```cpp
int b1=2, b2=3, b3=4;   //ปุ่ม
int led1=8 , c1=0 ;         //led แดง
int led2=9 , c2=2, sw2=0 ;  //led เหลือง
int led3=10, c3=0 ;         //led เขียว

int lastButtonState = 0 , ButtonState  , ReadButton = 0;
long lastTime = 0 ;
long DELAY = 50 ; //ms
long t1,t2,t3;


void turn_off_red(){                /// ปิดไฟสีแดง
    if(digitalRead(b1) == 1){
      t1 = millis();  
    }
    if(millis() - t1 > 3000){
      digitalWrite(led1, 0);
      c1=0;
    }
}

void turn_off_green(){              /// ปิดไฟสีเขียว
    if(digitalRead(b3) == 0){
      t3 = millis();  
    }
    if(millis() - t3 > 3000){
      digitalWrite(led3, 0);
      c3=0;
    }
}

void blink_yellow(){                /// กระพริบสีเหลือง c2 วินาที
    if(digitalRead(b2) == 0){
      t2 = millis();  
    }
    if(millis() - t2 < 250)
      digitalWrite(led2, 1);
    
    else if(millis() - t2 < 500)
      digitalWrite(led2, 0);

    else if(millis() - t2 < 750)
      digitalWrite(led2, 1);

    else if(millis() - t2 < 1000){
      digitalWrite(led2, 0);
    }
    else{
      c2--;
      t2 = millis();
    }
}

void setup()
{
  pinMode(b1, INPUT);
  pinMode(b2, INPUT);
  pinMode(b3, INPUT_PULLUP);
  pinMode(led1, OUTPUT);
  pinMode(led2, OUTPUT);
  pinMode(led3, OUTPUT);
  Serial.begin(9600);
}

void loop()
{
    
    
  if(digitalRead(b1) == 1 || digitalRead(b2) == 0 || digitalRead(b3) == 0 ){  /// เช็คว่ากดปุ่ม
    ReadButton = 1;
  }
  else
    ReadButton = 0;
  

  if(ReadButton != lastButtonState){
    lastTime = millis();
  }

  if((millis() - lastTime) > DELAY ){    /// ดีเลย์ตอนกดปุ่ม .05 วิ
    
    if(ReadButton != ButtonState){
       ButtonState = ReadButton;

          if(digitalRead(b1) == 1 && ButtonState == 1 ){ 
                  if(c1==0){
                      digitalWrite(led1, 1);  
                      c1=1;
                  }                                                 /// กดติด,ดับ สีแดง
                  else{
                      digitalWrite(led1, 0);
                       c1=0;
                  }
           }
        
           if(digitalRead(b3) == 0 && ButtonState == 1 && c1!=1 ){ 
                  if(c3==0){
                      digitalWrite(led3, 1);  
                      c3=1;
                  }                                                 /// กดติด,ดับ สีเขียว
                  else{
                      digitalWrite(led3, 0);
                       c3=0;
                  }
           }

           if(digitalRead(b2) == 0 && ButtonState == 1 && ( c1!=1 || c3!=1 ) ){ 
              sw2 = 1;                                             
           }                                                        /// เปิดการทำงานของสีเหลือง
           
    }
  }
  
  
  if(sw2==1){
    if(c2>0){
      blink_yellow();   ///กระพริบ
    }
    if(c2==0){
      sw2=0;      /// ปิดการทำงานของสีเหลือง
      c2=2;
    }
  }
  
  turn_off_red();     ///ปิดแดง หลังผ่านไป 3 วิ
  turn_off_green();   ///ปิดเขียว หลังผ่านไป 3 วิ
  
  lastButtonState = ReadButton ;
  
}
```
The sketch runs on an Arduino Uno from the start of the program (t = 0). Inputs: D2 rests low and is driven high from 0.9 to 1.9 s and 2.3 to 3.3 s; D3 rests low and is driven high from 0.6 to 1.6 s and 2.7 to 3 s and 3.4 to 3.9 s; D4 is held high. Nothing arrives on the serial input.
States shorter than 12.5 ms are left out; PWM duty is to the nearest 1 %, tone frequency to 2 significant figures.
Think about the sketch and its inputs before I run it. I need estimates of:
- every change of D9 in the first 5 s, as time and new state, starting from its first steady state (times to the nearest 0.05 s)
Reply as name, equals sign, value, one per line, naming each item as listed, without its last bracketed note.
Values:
every change of D9 in the first 5 s, as time and new state, starting from its first steady state = 0 s low; 0.05 s high; 0.85 s low; 1.1 s high; 1.35 s low; 1.6 s high; 2.95 s low; 3 s high; 3.65 s low; 3.9 s high
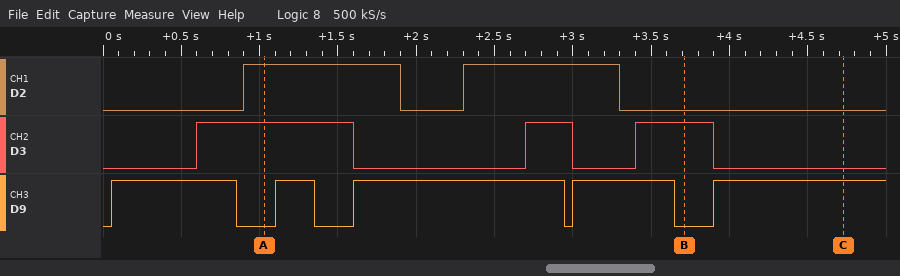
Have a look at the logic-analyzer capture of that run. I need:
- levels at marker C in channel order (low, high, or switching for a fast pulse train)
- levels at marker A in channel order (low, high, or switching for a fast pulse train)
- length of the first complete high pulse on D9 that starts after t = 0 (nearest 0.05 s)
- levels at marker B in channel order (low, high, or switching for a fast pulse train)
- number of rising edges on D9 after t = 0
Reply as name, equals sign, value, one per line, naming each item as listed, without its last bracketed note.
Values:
levels at marker C in channel order = D2 low, D3 low, D9 high
levels at marker A in channel order = D2 high, D3 high, D9 low
length of the first complete high pulse on D9 that starts after t = 0 = 0.80 s
levels at marker B in channel order = D2 low, D3 high, D9 low
number of rising edges on D9 after t = 0 = 5
